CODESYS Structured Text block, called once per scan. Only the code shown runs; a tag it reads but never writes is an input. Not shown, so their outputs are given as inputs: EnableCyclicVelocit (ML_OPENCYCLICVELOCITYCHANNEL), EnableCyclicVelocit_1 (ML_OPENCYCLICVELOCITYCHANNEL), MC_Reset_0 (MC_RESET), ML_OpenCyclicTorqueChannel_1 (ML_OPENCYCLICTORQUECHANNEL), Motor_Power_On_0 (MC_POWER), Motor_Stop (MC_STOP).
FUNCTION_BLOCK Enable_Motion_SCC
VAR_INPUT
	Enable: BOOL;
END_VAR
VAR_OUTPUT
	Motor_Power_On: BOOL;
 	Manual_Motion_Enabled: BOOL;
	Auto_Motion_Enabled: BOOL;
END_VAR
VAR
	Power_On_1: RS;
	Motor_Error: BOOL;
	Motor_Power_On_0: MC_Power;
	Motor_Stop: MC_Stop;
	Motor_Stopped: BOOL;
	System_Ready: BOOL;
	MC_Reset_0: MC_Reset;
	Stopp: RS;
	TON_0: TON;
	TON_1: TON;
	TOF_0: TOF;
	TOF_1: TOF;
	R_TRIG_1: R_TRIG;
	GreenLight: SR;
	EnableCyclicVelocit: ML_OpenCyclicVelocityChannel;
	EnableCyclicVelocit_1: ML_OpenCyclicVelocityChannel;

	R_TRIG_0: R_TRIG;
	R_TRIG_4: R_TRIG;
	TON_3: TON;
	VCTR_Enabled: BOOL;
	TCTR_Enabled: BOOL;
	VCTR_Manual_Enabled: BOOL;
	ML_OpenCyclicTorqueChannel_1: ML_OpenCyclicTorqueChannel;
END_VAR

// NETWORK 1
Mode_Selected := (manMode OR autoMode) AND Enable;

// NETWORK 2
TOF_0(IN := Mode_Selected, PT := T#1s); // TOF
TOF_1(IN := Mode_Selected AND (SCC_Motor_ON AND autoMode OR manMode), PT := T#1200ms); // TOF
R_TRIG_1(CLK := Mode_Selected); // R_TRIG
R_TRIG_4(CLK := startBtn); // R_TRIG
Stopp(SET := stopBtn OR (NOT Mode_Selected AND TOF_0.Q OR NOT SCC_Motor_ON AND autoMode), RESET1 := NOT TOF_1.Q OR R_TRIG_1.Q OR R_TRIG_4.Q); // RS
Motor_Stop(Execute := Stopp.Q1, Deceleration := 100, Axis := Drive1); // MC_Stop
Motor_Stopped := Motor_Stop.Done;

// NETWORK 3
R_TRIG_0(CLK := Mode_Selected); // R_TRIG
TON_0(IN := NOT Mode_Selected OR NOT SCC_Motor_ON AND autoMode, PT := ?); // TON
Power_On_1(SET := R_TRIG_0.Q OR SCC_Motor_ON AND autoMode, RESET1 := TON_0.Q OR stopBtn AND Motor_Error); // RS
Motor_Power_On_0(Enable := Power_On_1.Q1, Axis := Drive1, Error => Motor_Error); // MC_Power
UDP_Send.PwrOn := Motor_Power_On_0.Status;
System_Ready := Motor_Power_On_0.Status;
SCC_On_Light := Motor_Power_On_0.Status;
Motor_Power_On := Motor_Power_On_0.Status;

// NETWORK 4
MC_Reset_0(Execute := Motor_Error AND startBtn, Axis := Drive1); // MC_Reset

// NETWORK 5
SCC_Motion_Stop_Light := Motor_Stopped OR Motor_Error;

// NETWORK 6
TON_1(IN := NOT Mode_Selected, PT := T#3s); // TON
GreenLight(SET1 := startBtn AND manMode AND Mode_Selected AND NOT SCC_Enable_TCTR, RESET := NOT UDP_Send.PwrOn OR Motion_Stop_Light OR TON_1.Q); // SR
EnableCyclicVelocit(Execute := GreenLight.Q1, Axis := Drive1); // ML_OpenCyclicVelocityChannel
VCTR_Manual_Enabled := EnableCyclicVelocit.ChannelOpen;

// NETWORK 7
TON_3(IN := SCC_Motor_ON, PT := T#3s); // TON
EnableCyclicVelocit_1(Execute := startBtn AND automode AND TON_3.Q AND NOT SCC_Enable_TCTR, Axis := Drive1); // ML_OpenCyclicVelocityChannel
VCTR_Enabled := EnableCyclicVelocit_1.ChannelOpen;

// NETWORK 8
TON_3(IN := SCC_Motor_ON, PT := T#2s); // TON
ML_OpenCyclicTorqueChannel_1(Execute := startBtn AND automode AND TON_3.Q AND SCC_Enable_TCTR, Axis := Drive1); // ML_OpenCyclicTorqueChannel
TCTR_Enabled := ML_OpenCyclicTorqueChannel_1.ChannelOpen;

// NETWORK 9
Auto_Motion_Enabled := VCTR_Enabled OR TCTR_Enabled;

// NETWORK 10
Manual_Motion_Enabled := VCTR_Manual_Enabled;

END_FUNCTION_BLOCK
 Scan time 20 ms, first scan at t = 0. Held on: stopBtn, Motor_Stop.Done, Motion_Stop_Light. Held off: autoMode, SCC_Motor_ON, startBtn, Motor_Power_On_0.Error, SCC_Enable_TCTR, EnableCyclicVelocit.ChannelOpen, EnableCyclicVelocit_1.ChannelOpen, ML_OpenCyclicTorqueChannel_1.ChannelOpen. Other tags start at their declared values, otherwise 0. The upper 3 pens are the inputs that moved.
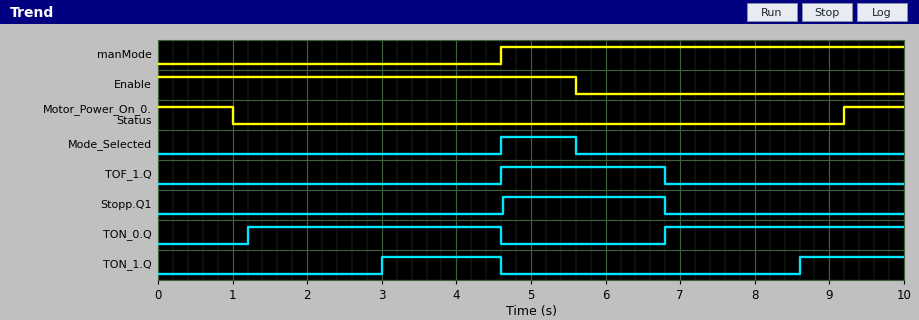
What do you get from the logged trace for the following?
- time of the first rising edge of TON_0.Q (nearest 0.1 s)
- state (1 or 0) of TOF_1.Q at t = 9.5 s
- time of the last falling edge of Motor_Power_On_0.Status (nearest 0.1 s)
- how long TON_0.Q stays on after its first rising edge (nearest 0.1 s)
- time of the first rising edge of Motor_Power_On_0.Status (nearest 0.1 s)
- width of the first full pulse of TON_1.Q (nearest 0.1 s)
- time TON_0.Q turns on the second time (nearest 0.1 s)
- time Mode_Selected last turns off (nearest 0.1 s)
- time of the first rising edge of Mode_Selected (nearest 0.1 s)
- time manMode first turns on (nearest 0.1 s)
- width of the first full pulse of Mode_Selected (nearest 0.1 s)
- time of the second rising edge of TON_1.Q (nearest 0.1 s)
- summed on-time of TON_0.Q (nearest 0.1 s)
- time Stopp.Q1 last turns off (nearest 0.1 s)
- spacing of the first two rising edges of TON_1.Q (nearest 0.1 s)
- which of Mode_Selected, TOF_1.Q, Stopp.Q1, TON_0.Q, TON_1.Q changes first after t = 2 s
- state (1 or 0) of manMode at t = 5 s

1.2 s
0
1.0 s
3.4 s
9.2 s
1.6 s
6.8 s
5.6 s
4.6 s
4.6 s
1.0 s
8.6 s
6.6 s
6.8 s
5.6 s
TON_1.Q
1
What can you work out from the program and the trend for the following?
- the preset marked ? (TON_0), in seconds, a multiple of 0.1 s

1.2 s
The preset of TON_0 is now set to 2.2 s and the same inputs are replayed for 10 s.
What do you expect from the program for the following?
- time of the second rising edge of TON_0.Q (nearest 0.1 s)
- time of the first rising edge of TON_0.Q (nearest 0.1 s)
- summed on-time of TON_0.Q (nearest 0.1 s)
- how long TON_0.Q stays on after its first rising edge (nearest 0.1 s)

7.8 s
2.2 s
4.6 s
2.4 s
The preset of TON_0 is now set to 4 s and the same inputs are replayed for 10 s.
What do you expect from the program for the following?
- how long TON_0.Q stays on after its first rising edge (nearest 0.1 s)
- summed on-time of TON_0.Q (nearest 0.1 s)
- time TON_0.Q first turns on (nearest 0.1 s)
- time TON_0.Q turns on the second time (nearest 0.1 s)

0.6 s
1.0 s
4.0 s
9.6 s
